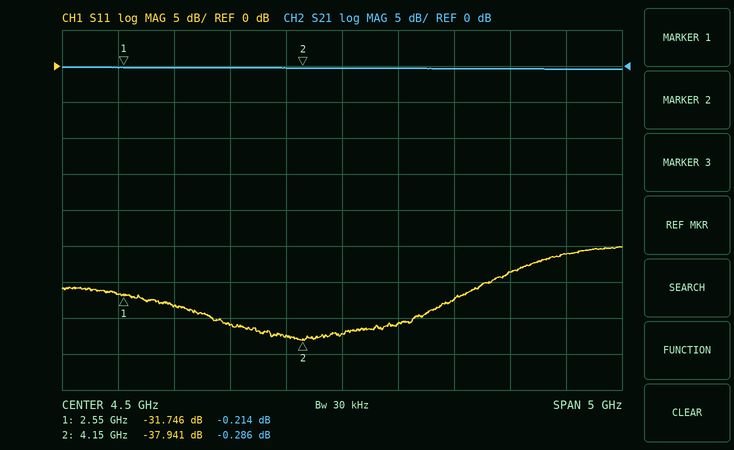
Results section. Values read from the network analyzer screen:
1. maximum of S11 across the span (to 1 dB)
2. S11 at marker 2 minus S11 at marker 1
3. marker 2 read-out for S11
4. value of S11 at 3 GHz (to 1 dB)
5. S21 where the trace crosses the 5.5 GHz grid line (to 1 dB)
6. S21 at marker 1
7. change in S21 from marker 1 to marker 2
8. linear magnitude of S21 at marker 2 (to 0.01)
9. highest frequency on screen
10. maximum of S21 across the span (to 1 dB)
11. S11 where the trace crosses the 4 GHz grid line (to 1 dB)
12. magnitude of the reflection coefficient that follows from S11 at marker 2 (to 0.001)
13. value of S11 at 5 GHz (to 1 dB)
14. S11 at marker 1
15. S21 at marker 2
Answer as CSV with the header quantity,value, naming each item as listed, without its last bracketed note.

quantity,value
maximum of S11 across the span,-25 dB
S11 at marker 2 minus S11 at marker 1,-6.195 dB
marker 2 read-out for S11,-37.941 dB
value of S11 at 3 GHz,-33 dB
S21 where the trace crosses the 5.5 GHz grid line,0 dB
S21 at marker 1,-0.214 dB
change in S21 from marker 1 to marker 2,-0.072 dB
linear magnitude of S21 at marker 2,0.97
highest frequency on screen,7 GHz
maximum of S21 across the span,0 dB
S11 where the trace crosses the 4 GHz grid line,-37 dB
magnitude of the reflection coefficient that follows from S11 at marker 2,0.013
value of S11 at 5 GHz,-36 dB
S11 at marker 1,-31.746 dB
S21 at marker 2,-0.286 dB
